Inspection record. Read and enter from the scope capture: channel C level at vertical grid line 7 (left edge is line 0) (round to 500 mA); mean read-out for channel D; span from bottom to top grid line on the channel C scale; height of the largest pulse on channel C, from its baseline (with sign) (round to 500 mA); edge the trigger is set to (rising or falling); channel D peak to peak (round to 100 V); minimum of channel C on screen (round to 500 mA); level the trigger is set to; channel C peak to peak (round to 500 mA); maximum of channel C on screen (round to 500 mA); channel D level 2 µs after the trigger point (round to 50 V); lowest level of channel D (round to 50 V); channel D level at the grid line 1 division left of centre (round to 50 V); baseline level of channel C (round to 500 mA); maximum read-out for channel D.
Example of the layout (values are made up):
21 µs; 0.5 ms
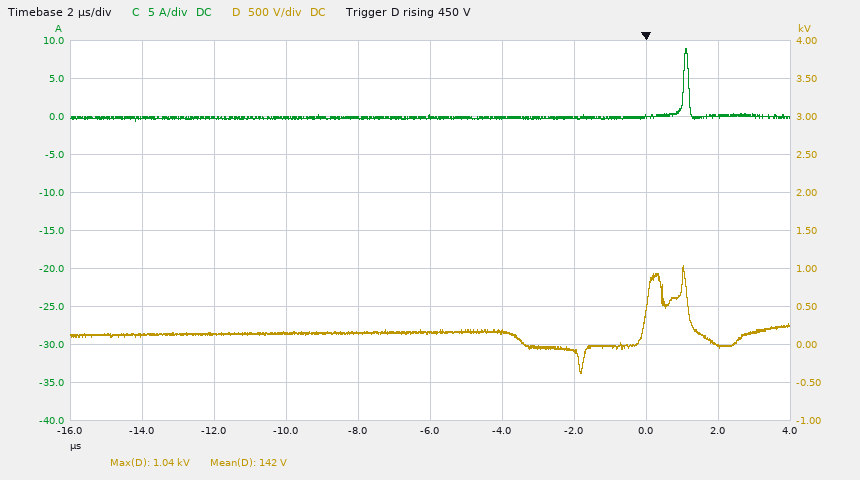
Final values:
0.0 A; 142 V; 50 A; +9.0 A; rising; 1.40 kV; -500 mA; 450 V; 9.5 A; 9.0 A; 0 V; -400 V; 150 V; 0.0 A; 1.04 kV
